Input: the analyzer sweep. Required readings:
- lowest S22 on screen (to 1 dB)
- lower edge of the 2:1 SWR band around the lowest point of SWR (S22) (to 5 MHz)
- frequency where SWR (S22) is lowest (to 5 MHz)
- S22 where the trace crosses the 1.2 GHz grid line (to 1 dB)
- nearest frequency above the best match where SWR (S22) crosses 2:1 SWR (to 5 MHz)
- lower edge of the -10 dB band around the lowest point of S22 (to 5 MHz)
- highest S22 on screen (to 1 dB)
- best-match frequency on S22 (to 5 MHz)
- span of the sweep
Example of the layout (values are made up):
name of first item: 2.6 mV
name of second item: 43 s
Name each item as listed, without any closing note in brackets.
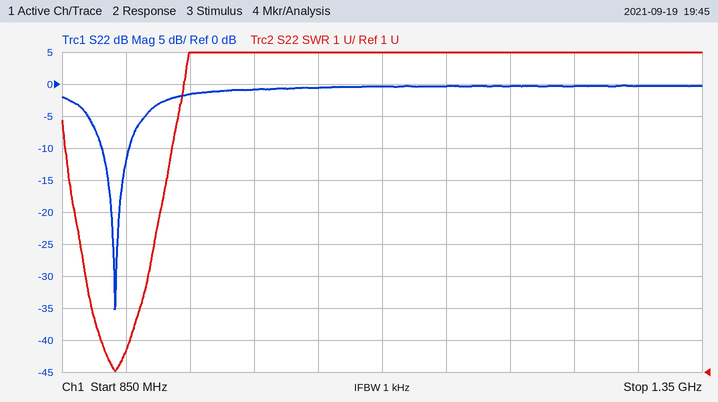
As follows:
lowest S22 on screen: -35 dB
lower edge of the 2:1 SWR band around the lowest point of SWR (S22): 880 MHz
frequency where SWR (S22) is lowest: 890 MHz
S22 where the trace crosses the 1.2 GHz grid line: 0 dB
nearest frequency above the best match where SWR (S22) crosses 2:1 SWR: 905 MHz
lower edge of the -10 dB band around the lowest point of S22: 880 MHz
highest S22 on screen: 0 dB
best-match frequency on S22: 890 MHz
span of the sweep: 500 MHz
